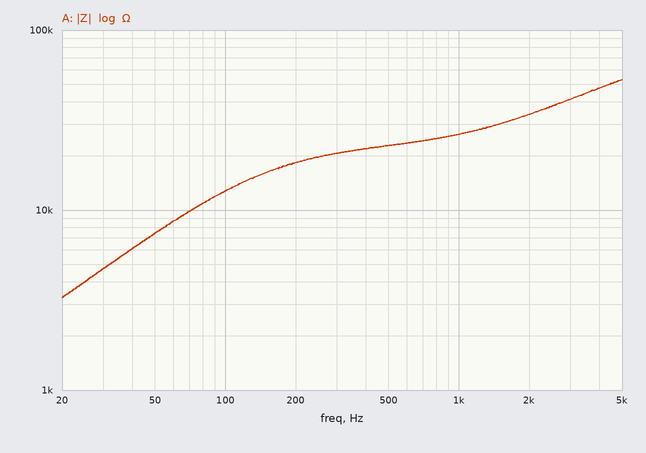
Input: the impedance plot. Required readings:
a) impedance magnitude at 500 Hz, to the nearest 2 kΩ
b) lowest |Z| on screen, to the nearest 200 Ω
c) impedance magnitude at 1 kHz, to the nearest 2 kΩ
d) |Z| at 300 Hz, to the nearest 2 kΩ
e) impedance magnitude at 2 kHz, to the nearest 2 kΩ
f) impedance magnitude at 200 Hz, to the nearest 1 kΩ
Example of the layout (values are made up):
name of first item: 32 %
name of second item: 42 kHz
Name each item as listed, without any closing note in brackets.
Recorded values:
impedance magnitude at 500 Hz, to the nearest 2 kΩ: 22 kΩ
lowest |Z| on screen, to the nearest 200 Ω: 3.2 kΩ
impedance magnitude at 1 kHz, to the nearest 2 kΩ: 26 kΩ
|Z| at 300 Hz, to the nearest 2 kΩ: 20 kΩ
impedance magnitude at 2 kHz, to the nearest 2 kΩ: 34 kΩ
impedance magnitude at 200 Hz, to the nearest 1 kΩ: 18 kΩ
